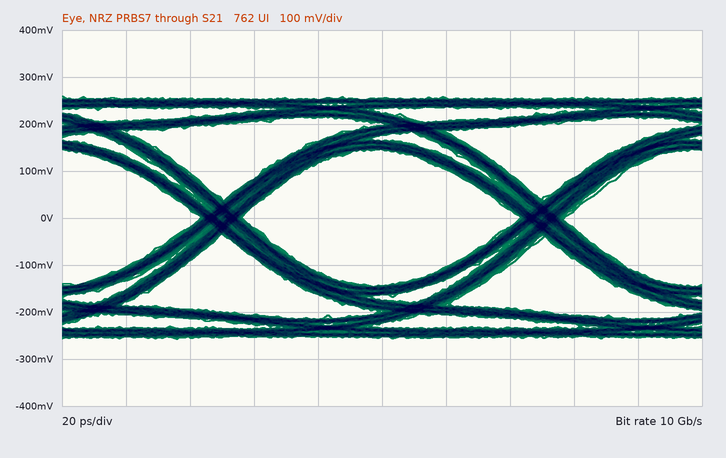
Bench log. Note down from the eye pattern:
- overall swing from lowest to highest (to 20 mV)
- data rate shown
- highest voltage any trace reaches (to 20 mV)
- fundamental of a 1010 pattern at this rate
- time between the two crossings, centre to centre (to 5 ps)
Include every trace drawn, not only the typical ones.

520 mV
10 Gb/s
260 mV
5 GHz
100 ps
